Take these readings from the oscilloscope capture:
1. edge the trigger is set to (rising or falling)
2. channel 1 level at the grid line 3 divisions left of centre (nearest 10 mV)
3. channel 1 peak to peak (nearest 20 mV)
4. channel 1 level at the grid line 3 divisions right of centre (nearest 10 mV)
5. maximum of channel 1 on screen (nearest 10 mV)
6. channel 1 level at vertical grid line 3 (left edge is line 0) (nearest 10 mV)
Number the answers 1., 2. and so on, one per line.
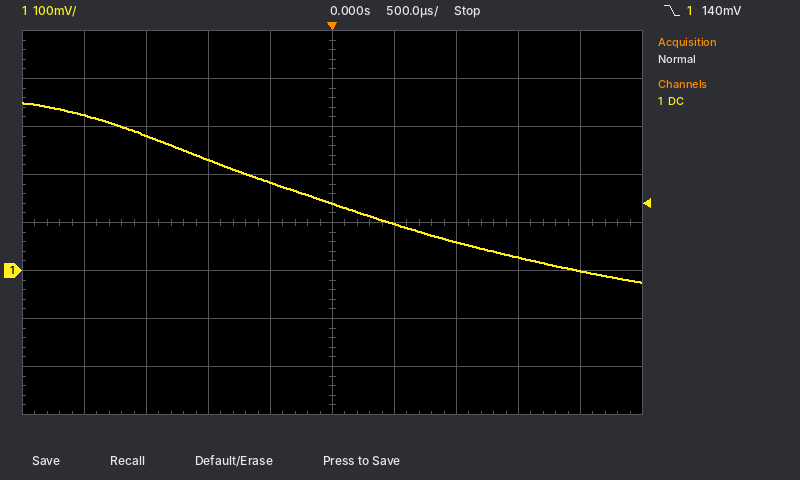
1. falling
2. 280 mV
3. 380 mV
4. 30 mV
5. 350 mV
6. 230 mV
